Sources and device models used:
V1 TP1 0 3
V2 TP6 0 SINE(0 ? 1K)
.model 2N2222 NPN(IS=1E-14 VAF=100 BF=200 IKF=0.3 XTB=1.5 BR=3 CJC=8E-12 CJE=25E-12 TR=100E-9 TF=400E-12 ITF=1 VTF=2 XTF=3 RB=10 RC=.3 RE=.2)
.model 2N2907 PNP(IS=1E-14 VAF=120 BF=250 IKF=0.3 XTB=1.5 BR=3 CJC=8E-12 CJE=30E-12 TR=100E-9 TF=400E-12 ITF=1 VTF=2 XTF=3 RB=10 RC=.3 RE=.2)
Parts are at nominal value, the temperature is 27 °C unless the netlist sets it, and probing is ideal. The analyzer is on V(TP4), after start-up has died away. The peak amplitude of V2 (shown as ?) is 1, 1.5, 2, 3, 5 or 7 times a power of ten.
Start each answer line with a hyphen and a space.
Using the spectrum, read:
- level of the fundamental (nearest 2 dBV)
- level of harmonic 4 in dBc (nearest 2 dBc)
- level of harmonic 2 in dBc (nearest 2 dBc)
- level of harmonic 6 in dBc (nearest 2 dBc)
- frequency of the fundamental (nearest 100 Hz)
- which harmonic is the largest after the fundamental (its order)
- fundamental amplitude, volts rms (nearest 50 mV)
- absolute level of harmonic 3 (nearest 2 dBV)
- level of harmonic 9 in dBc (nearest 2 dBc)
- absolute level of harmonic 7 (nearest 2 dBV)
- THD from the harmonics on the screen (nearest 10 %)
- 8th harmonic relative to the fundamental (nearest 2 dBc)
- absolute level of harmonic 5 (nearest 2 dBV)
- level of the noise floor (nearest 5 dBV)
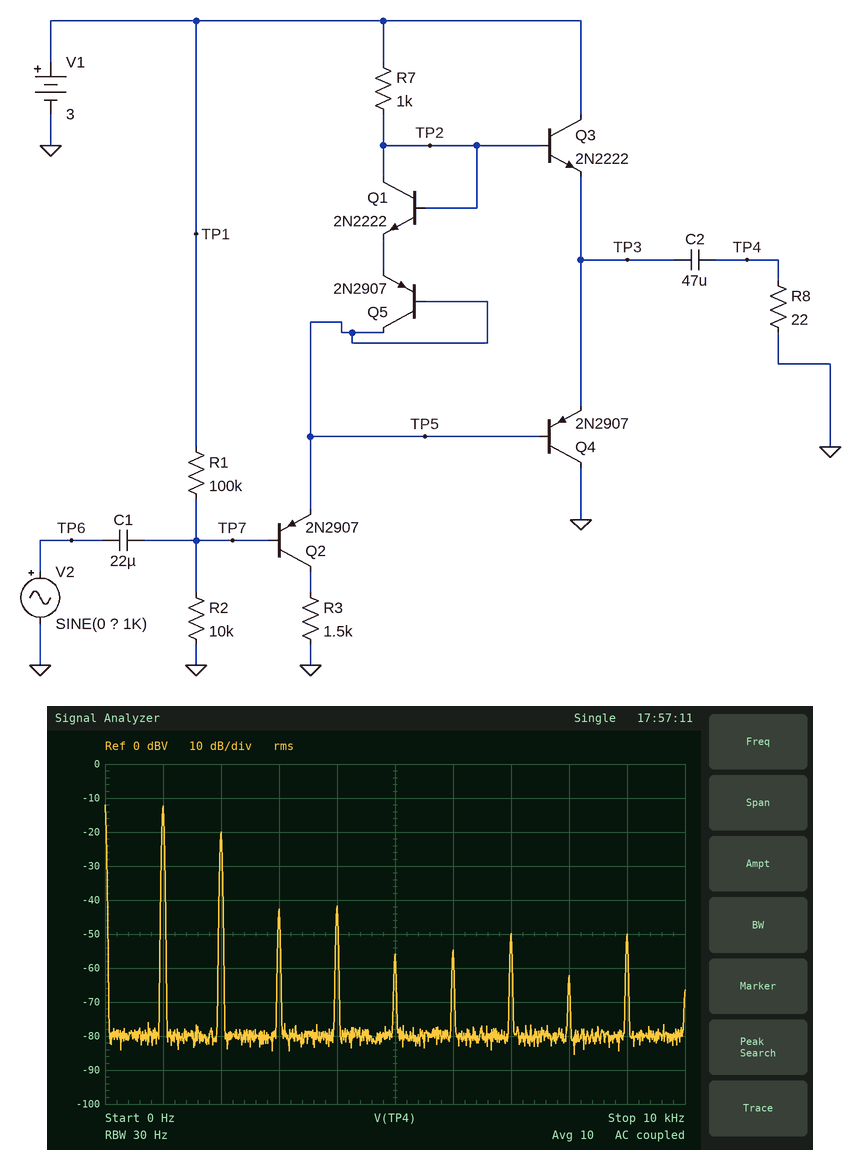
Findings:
- -12 dBV
- -30 dBc
- -8 dBc
- -42 dBc
- 1.0 kHz
- 2
- 250 mV
- -42 dBV
- -38 dBc
- -50 dBV
- 40 %
- -50 dBc
- -56 dBV
- -80 dBV
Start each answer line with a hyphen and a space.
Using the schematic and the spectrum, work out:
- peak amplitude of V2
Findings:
- 1 V
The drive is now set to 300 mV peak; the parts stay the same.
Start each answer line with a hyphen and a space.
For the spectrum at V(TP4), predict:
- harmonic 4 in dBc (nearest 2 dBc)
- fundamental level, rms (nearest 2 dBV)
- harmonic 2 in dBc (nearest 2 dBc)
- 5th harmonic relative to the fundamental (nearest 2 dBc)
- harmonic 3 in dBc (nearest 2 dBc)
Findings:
- -52 dBc
- -18 dBV
- -30 dBc
- -36 dBc
- -28 dBc
